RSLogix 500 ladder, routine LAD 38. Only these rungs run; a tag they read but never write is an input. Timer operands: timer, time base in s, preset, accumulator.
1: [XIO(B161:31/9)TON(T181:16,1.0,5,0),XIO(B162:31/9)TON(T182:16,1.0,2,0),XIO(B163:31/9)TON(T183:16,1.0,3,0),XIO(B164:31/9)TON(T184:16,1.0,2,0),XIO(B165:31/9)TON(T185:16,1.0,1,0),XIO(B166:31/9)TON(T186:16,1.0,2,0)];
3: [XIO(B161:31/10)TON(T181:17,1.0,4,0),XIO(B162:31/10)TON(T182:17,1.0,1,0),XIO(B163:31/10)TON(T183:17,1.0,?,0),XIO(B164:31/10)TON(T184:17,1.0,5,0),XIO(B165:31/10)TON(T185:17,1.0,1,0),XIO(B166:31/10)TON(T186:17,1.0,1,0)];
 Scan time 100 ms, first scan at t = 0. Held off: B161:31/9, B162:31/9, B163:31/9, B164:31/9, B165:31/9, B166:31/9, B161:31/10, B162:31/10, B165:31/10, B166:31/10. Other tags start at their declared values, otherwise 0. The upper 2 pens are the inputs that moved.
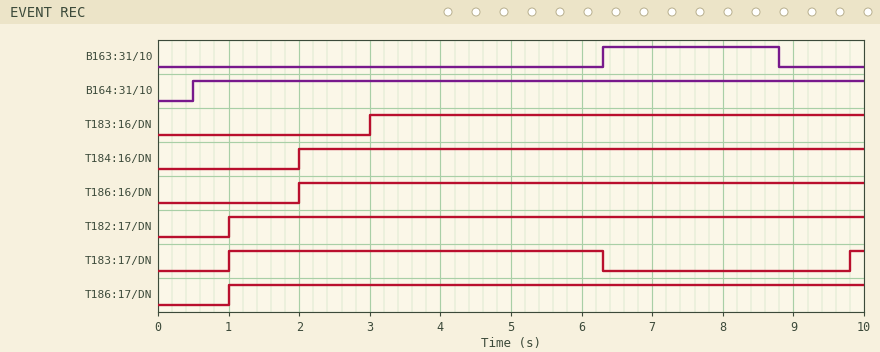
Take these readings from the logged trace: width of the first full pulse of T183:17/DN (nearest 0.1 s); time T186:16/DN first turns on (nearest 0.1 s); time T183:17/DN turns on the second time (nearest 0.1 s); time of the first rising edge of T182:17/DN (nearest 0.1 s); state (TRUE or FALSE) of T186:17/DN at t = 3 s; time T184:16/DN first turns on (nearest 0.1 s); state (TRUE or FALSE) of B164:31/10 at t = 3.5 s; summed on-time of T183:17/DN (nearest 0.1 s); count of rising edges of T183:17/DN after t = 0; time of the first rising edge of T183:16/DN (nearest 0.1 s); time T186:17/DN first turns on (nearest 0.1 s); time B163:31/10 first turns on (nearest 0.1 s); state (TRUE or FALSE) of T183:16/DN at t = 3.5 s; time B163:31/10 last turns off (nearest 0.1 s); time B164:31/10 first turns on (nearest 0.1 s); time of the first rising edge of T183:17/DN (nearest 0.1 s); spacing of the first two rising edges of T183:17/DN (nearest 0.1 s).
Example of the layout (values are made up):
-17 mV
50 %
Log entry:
5.3 s
2.0 s
9.8 s
1.0 s
TRUE
2.0 s
TRUE
5.5 s
2
3.0 s
1.0 s
6.3 s
TRUE
8.8 s
0.5 s
1.0 s
8.8 s
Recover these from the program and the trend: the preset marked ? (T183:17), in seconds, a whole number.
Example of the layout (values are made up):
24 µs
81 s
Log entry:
1 s
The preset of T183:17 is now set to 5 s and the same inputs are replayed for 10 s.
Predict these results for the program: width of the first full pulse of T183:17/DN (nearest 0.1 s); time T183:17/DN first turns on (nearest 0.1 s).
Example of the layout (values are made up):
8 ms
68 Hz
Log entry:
1.3 s
5.0 s
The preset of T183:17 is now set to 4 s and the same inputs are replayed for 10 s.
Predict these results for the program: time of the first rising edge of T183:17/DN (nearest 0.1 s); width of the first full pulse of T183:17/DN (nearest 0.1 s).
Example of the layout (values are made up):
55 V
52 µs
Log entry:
4.0 s
2.3 s
